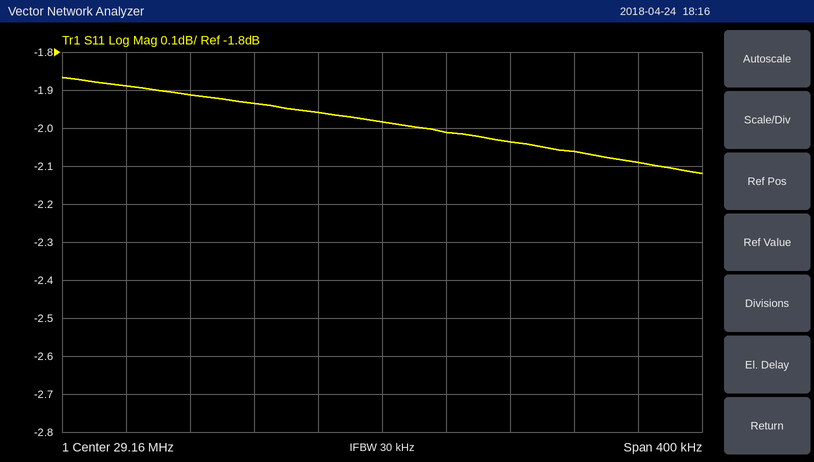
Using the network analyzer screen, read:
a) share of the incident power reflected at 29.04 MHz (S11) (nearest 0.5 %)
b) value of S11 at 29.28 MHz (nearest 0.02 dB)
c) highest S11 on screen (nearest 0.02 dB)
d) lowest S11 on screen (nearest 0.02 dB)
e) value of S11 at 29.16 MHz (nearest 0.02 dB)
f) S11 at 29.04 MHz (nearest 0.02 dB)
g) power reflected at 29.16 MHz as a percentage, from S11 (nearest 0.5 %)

64.5 %
-2.06 dB
-1.86 dB
-2.12 dB
-1.98 dB
-1.92 dB
63.5 %
